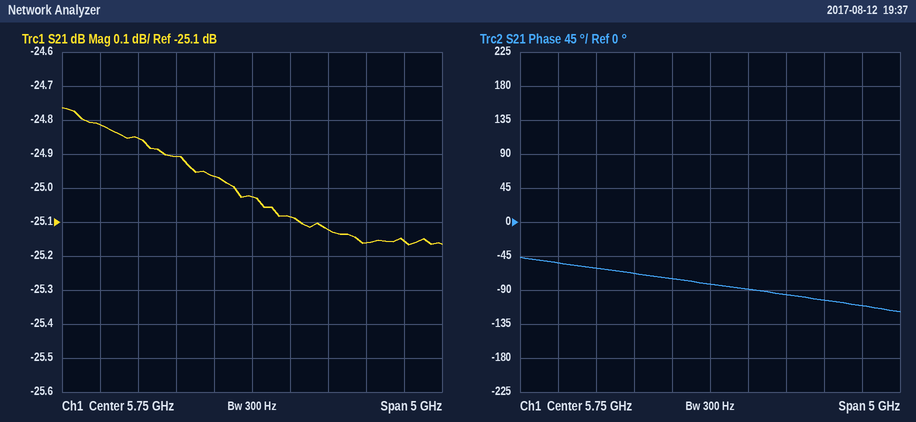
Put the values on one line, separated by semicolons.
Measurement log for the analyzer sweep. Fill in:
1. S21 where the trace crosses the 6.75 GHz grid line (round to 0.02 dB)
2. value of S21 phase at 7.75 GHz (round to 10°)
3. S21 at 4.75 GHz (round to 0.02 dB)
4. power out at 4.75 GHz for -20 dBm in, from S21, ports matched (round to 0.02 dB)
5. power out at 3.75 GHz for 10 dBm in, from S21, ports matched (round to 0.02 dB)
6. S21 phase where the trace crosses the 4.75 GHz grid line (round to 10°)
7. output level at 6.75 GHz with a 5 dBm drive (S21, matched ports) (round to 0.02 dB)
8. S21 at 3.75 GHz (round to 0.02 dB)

-25.12 dB; -110°; -24.90 dB; -44.90 dBm; -14.82 dBm; -70°; -20.12 dBm; -24.82 dB
